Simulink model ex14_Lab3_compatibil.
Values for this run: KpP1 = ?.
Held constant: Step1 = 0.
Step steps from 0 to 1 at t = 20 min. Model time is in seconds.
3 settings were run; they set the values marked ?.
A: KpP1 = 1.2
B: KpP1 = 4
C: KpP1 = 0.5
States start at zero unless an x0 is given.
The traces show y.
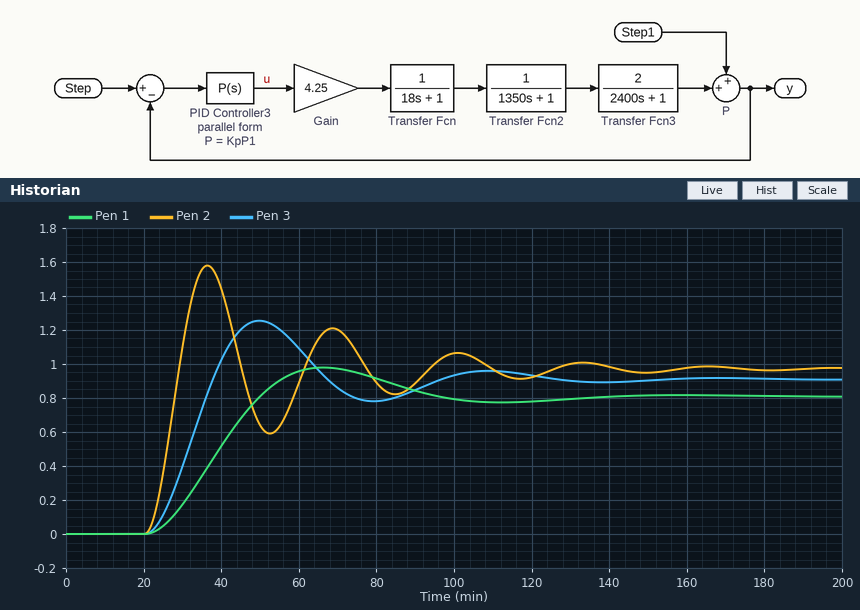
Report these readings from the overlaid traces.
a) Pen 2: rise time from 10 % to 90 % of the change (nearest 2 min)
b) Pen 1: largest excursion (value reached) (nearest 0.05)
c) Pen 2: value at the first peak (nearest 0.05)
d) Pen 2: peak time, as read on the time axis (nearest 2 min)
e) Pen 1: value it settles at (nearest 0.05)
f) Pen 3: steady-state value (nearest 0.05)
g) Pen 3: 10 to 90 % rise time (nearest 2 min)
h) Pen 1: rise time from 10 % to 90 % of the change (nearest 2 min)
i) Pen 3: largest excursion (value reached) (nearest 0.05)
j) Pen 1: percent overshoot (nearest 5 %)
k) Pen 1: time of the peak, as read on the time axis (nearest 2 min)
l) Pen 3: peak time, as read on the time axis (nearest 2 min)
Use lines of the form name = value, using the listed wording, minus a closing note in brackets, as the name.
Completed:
Pen 2: rise time from 10 % to 90 % of the change = 6 min
Pen 1: largest excursion (value reached) = 1.00
Pen 2: value at the first peak = 1.60
Pen 2: peak time, as read on the time axis = 36 min
Pen 1: value it settles at = 0.80
Pen 3: steady-state value = 0.90
Pen 3: 10 to 90 % rise time = 12 min
Pen 1: rise time from 10 % to 90 % of the change = 20 min
Pen 3: largest excursion (value reached) = 1.25
Pen 1: percent overshoot = 20 %
Pen 1: time of the peak, as read on the time axis = 66 min
Pen 3: peak time, as read on the time axis = 50 min
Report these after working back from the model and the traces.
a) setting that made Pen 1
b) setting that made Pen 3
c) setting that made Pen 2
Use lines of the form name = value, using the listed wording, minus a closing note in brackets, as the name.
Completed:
setting that made Pen 1 = C
setting that made Pen 3 = A
setting that made Pen 2 = B
